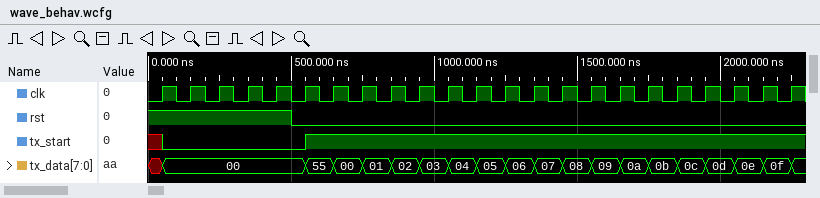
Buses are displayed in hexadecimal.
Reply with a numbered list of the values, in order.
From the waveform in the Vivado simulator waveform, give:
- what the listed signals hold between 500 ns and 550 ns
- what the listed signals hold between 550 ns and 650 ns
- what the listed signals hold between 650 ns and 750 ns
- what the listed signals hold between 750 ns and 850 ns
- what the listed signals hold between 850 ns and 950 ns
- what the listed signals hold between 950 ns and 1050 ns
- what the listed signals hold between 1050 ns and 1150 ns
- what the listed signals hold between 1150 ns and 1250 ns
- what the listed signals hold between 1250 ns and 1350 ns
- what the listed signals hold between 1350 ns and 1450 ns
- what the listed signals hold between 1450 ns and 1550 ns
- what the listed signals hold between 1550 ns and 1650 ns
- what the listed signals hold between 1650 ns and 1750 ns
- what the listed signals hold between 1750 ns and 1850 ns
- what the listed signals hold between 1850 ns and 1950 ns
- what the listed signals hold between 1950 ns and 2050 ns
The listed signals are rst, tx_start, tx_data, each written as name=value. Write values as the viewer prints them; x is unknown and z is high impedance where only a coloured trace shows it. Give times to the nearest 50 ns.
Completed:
1. rst=0, tx_start=0, tx_data=00
2. rst=0, tx_start=1, tx_data=55
3. rst=0, tx_start=1, tx_data=00
4. rst=0, tx_start=1, tx_data=01
5. rst=0, tx_start=1, tx_data=02
6. rst=0, tx_start=1, tx_data=03
7. rst=0, tx_start=1, tx_data=04
8. rst=0, tx_start=1, tx_data=05
9. rst=0, tx_start=1, tx_data=06
10. rst=0, tx_start=1, tx_data=07
11. rst=0, tx_start=1, tx_data=08
12. rst=0, tx_start=1, tx_data=09
13. rst=0, tx_start=1, tx_data=0a
14. rst=0, tx_start=1, tx_data=0b
15. rst=0, tx_start=1, tx_data=0c
16. rst=0, tx_start=1, tx_data=0d
